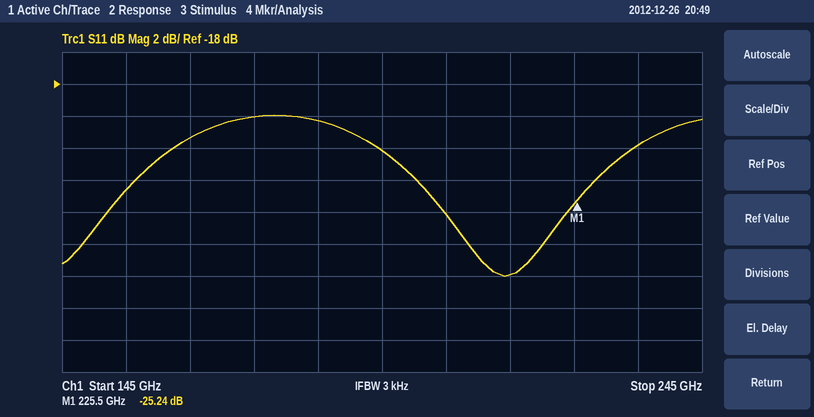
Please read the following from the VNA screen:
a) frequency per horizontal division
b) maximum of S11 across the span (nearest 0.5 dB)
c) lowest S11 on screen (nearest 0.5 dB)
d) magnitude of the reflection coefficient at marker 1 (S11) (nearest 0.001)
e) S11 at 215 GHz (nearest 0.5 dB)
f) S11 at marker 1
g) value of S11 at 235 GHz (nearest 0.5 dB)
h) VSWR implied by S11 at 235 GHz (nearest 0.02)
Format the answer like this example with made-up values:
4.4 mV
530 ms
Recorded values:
10 GHz
-20.0 dB
-30.0 dB
0.055
-30.0 dB
-25.24 dB
-22.0 dB
1.18
